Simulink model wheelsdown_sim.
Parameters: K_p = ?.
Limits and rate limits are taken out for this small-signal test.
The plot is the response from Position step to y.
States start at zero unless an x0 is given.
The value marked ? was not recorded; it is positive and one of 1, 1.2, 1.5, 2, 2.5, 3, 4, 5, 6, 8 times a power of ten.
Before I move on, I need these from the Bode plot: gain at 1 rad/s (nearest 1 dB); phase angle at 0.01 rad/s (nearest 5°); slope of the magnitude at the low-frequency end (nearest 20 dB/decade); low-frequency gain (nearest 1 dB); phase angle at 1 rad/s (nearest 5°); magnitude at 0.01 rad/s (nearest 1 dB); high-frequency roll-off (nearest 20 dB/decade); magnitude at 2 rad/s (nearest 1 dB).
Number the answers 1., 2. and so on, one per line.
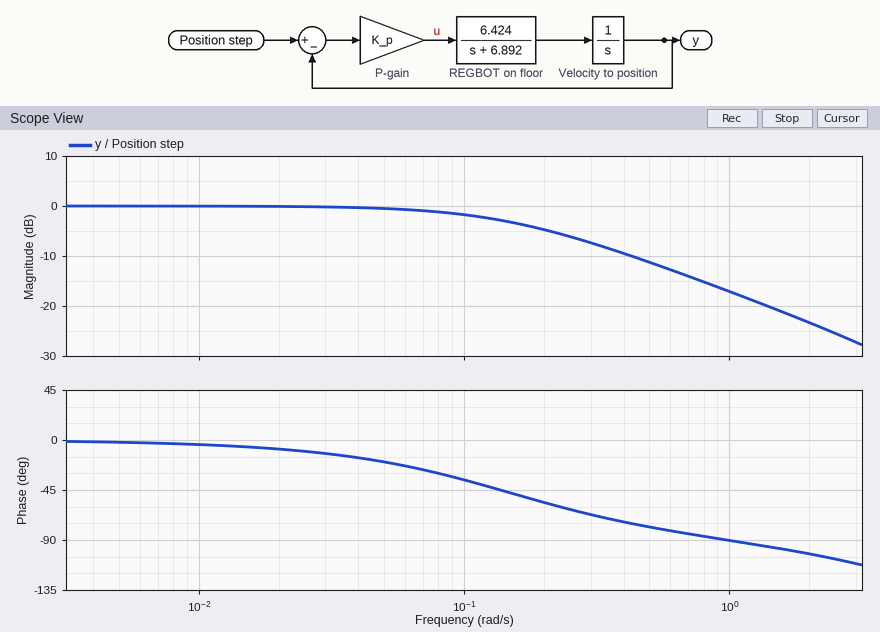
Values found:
1. -17 dB
2. -5°
3. 0 dB/decade
4. 0 dB
5. -90°
6. 0 dB
7. -20 dB/decade
8. -23 dB
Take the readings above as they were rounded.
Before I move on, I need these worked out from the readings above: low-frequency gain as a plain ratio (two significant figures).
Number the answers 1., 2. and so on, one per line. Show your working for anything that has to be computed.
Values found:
1. 10^(0 / 20) = 1.0
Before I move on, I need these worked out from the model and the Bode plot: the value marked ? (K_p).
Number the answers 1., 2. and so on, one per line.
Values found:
1. 0.15
